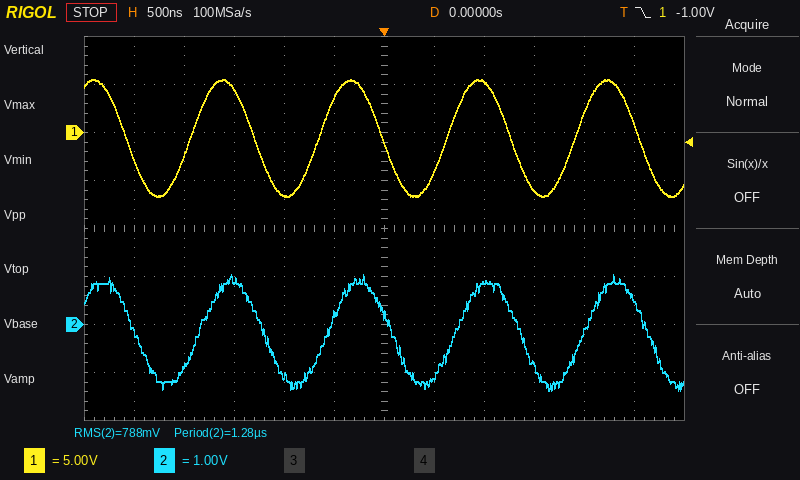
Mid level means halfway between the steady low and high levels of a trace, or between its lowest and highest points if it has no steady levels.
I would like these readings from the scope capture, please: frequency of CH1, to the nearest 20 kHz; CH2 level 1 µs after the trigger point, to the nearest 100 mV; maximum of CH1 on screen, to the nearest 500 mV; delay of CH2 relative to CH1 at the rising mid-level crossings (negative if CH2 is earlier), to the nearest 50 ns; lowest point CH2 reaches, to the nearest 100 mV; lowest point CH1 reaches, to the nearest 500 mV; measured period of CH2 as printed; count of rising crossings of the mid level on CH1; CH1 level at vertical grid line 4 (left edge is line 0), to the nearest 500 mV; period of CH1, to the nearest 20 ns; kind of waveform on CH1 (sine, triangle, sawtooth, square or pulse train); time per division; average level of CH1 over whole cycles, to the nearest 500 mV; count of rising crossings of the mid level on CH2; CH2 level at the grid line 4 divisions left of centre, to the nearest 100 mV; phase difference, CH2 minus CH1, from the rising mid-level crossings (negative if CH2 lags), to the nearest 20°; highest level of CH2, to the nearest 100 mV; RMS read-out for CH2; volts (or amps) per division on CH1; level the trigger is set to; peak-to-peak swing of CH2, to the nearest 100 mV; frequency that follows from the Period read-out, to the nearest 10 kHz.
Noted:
780 kHz
900 mV
5.5 V
+100 ns
-1.4 V
-6.5 V
1.28 µs
4
-6.5 V
1.28 µs
sine
500 ns
-500 mV
4
-900 mV
-20°
1.0 V
788 mV
5 V
-1.00 V
2.4 V
780 kHz
